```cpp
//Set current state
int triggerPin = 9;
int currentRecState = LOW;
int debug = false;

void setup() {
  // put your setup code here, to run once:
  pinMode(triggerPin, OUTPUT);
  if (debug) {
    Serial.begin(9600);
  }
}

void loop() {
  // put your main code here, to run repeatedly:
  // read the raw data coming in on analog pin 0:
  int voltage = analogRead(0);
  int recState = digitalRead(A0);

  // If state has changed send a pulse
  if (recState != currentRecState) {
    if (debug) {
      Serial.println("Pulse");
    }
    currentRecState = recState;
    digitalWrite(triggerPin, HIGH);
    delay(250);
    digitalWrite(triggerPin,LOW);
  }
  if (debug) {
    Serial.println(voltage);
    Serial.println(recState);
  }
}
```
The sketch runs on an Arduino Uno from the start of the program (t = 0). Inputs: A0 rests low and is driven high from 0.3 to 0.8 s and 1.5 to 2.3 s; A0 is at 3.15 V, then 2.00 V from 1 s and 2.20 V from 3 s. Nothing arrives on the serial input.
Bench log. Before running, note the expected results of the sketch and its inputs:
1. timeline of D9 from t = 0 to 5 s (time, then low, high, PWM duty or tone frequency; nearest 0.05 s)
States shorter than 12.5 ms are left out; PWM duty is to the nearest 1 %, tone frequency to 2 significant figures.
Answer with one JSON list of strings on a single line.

["0 s low; 0.3 s high; 0.55 s low; 0.8 s high; 1.05 s low; 1.5 s high; 1.75 s low; 2.3 s high; 2.55 s low"]
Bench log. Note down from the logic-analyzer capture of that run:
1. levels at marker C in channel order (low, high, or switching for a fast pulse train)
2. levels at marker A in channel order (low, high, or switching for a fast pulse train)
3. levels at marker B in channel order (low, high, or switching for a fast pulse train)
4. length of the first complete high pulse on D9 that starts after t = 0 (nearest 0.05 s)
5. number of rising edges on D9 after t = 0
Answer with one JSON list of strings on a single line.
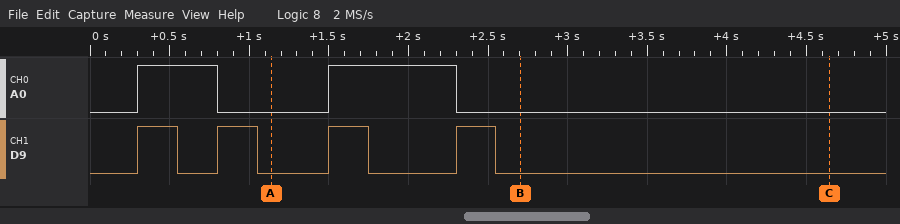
["A0 low, D9 low", "A0 low, D9 low", "A0 low, D9 low", "0.25 s", "4"]
